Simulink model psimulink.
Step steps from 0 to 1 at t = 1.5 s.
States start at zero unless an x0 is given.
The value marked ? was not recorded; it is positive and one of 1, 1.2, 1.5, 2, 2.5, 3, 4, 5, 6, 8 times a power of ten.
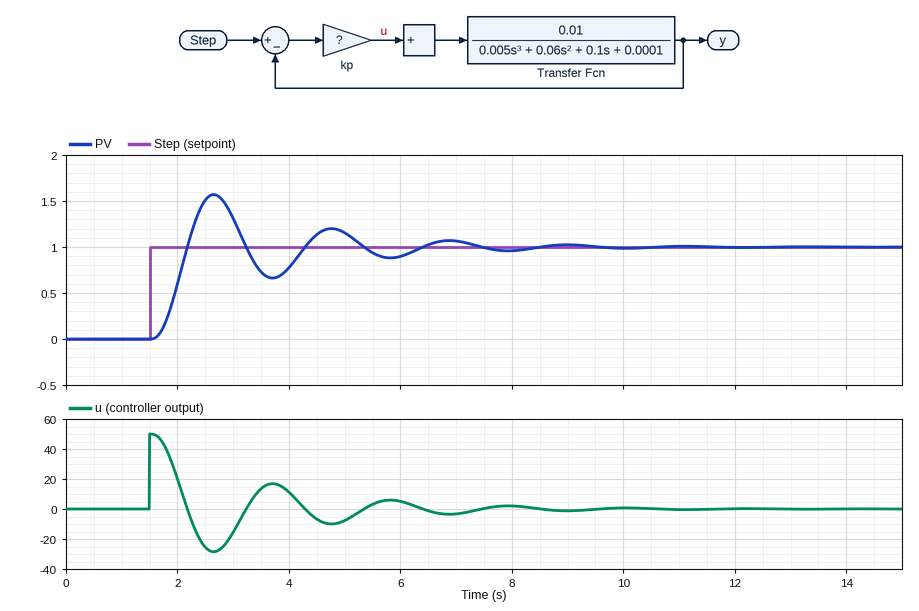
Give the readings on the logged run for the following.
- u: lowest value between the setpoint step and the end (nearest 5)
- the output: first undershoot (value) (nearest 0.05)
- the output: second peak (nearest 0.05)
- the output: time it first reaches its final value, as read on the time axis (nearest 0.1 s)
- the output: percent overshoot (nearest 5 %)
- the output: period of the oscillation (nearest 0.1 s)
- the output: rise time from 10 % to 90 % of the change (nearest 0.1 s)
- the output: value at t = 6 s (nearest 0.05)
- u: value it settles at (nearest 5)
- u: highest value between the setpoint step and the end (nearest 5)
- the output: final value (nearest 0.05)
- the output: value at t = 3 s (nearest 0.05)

-30
0.65
1.20
2.2 s
55 %
2.1 s
0.4 s
0.90
0
50
1.00
1.30
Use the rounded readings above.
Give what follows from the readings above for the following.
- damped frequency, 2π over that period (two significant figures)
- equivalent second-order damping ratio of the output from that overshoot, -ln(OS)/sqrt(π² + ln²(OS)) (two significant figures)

3.0 rad/s
0.19
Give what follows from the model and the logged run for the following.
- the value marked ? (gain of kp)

50
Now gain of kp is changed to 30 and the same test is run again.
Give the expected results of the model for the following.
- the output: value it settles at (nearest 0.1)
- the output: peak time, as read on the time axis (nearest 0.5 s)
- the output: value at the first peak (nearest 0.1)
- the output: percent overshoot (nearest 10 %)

1.0
3.0 s
1.4
40 %
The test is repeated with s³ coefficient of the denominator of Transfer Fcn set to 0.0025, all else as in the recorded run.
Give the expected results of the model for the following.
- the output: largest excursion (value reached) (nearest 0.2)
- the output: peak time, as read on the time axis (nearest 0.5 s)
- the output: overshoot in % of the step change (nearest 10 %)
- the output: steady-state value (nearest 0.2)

1.4
2.5 s
50 %
1.0
